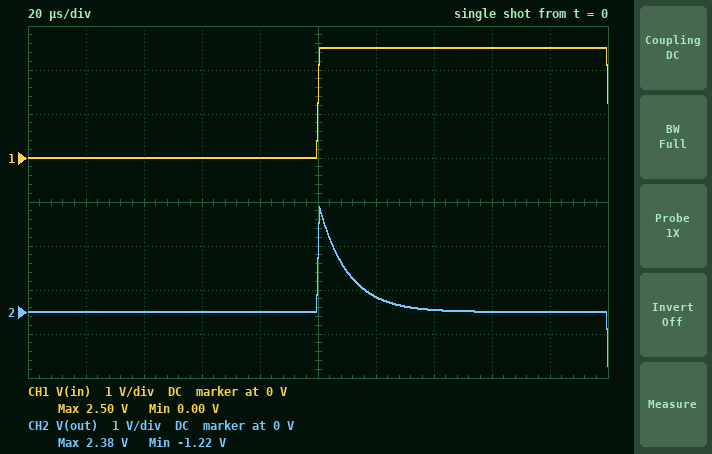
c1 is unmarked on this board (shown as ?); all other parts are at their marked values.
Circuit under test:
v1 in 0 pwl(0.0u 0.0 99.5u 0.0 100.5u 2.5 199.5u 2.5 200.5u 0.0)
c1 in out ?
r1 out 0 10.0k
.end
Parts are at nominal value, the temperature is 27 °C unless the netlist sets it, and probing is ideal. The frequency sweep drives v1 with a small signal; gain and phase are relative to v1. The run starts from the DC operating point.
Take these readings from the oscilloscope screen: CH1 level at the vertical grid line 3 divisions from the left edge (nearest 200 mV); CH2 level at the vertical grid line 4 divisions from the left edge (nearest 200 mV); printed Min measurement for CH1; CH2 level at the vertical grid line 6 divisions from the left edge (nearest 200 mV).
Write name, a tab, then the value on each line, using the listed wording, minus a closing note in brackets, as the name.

CH1 level at the vertical grid line 3 divisions from the left edge	0 V
CH2 level at the vertical grid line 4 divisions from the left edge	0 V
printed Min measurement for CH1	0.00 V
CH2 level at the vertical grid line 6 divisions from the left edge	400 mV
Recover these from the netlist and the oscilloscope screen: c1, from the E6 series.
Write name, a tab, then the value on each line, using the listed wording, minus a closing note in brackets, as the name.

c1, from the E6 series	1 nF
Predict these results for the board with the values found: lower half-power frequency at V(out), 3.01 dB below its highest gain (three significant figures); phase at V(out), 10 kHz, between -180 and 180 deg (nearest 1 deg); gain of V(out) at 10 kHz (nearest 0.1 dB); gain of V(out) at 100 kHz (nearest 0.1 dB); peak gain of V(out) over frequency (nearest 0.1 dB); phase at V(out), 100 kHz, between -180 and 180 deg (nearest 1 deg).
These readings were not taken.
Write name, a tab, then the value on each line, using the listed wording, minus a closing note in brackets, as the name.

lower half-power frequency at V(out), 3.01 dB below its highest gain	15.9 kHz
phase at V(out), 10 kHz, between -180 and 180 deg	58 deg
gain of V(out) at 10 kHz	-5.5 dB
gain of V(out) at 100 kHz	-0.1 dB
peak gain of V(out) over frequency	0 dB
phase at V(out), 100 kHz, between -180 and 180 deg	9 deg
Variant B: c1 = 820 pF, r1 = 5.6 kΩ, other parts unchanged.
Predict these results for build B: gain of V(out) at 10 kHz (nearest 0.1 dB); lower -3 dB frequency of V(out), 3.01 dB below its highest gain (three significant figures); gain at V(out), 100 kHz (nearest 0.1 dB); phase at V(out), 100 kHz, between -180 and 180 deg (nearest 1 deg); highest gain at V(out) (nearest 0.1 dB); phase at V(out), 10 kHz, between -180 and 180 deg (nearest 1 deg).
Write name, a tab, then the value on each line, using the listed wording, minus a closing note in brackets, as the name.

gain of V(out) at 10 kHz	-11.1 dB
lower -3 dB frequency of V(out), 3.01 dB below its highest gain	34.7 kHz
gain at V(out), 100 kHz	-0.5 dB
phase at V(out), 100 kHz, between -180 and 180 deg	19 deg
highest gain at V(out)	0 dB
phase at V(out), 10 kHz, between -180 and 180 deg	74 deg
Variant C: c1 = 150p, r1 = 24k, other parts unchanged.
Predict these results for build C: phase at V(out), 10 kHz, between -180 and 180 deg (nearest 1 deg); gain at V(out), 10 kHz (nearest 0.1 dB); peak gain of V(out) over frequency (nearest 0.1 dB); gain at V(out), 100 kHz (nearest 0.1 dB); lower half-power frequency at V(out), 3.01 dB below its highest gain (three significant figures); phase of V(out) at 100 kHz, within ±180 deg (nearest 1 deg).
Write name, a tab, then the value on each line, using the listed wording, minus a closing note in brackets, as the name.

phase at V(out), 10 kHz, between -180 and 180 deg	77 deg
gain at V(out), 10 kHz	-13.1 dB
peak gain of V(out) over frequency	0 dB
gain at V(out), 100 kHz	-0.8 dB
lower half-power frequency at V(out), 3.01 dB below its highest gain	44.2 kHz
phase of V(out) at 100 kHz, within ±180 deg	24 deg
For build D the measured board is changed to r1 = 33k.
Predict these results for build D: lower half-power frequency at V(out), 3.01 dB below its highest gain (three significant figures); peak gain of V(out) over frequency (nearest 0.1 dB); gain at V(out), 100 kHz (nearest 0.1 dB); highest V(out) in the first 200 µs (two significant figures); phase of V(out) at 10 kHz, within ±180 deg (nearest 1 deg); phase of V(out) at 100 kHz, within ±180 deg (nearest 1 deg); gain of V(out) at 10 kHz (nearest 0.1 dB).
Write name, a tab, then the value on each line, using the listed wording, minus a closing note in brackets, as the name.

lower half-power frequency at V(out), 3.01 dB below its highest gain	4.82 kHz
peak gain of V(out) over frequency	0 dB
gain at V(out), 100 kHz	0 dB
highest V(out) in the first 200 µs	2.5 V
phase of V(out) at 10 kHz, within ±180 deg	26 deg
phase of V(out) at 100 kHz, within ±180 deg	3 deg
gain of V(out) at 10 kHz	-0.9 dB
